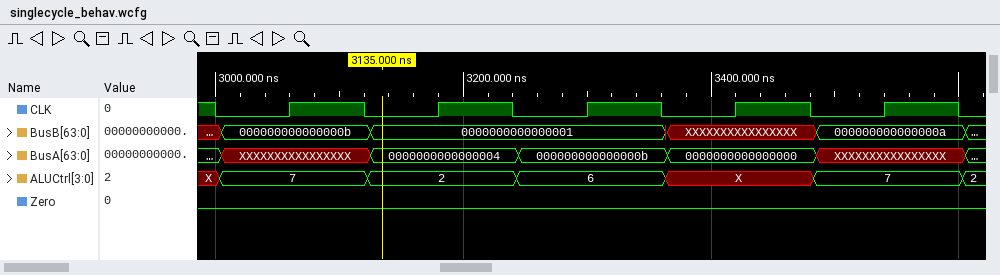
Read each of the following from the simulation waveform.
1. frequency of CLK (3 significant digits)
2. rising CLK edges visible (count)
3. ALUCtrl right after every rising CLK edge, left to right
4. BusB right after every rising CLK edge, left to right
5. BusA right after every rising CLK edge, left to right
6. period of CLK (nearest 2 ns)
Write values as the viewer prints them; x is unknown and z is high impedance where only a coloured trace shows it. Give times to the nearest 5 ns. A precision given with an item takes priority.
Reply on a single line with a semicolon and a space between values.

8.33 MHz; 5; 7, 2, 6, X, 7; 000000000000000b, 0000000000000001, 0000000000000001, XXXXXXXXXXXXXXXX, 000000000000000a; XXXXXXXXXXXXXXXX, 0000000000000004, 000000000000000b, 0000000000000000, XXXXXXXXXXXXXXXX; 120 ns
